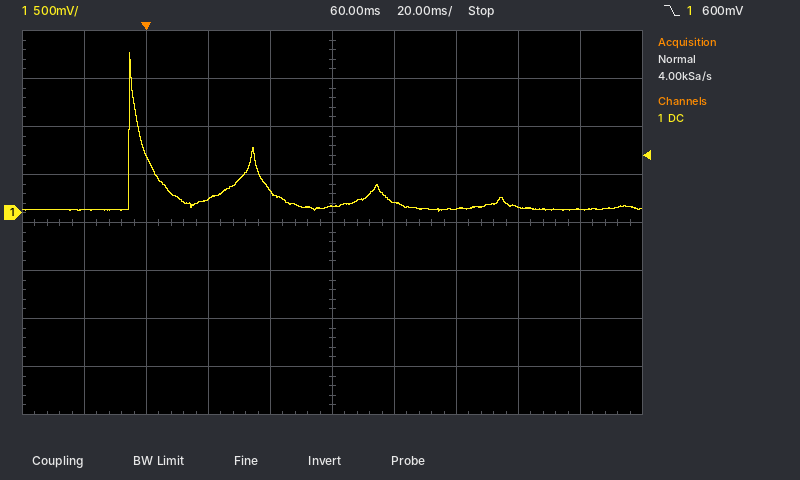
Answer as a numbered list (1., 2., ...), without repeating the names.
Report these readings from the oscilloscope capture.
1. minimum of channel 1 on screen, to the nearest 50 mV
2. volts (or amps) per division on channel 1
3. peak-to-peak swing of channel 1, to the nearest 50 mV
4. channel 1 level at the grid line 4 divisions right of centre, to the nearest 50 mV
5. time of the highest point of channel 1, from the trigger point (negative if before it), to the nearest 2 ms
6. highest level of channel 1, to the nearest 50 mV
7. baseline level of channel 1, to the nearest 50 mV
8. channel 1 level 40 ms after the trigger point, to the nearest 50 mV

1. 0 mV
2. 500 mV
3. 1.65 V
4. 50 mV
5. -6 ms
6. 1.65 V
7. 50 mV
8. 250 mV
